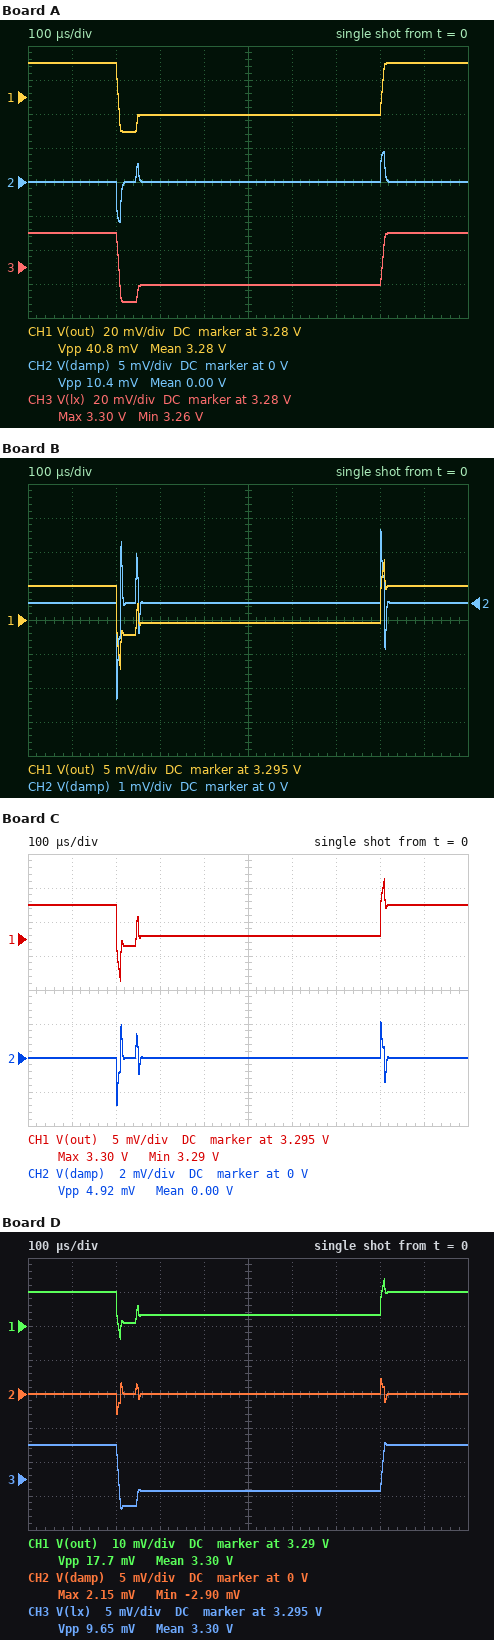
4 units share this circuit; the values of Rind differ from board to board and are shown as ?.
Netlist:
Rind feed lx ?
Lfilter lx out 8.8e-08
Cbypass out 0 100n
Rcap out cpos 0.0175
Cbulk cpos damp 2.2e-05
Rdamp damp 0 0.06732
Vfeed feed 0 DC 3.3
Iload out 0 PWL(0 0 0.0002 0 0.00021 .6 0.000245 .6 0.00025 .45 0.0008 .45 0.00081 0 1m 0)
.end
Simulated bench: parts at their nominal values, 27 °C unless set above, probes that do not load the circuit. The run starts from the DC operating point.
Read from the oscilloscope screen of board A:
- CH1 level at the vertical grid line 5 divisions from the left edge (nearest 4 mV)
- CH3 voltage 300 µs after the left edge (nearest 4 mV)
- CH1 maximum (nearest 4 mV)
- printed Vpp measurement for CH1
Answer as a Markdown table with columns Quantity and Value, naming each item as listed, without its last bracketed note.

| Quantity | Value |
|---|---|
| CH1 level at the vertical grid line 5 divisions from the left edge | 3.268 V |
| CH3 voltage 300 µs after the left edge | 3.268 V |
| CH1 maximum | 3.300 V |
| printed Vpp measurement for CH1 | 40.8 mV |
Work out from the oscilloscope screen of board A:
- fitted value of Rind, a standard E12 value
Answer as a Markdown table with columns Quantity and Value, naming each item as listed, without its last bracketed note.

| Quantity | Value |
|---|---|
| fitted value of Rind, a standard E12 value | 0.068 Ω |
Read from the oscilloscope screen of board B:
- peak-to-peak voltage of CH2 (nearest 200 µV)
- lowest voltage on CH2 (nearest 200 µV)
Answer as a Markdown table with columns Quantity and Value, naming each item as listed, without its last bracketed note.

| Quantity | Value |
|---|---|
| peak-to-peak voltage of CH2 | 5.0 mV |
| lowest voltage on CH2 | -2.8 mV |
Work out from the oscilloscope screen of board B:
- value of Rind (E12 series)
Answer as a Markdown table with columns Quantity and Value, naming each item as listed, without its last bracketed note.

| Quantity | Value |
|---|---|
| value of Rind | 0.012 Ω |
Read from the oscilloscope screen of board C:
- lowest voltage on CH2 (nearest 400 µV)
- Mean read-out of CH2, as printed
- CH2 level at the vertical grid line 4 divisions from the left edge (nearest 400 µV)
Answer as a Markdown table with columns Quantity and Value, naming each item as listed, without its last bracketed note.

| Quantity | Value |
|---|---|
| lowest voltage on CH2 | -2.8 mV |
| Mean read-out of CH2, as printed | 0.00 V |
| CH2 level at the vertical grid line 4 divisions from the left edge | 0 V |
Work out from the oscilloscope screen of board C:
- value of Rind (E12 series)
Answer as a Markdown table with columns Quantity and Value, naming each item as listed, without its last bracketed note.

| Quantity | Value |
|---|---|
| value of Rind | 0.01 Ω |
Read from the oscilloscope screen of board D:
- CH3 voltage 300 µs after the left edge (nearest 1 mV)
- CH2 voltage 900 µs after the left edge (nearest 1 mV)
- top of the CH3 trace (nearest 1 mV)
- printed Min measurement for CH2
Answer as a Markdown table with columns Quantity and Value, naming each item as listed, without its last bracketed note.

| Quantity | Value |
|---|---|
| CH3 voltage 300 µs after the left edge | 3.293 V |
| CH2 voltage 900 µs after the left edge | 0 V |
| top of the CH3 trace | 3.300 V |
| printed Min measurement for CH2 | -2.90 mV |
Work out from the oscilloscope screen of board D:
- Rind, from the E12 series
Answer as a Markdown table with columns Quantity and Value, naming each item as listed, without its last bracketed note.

| Quantity | Value |
|---|---|
| Rind, from the E12 series | 0.015 Ω |
